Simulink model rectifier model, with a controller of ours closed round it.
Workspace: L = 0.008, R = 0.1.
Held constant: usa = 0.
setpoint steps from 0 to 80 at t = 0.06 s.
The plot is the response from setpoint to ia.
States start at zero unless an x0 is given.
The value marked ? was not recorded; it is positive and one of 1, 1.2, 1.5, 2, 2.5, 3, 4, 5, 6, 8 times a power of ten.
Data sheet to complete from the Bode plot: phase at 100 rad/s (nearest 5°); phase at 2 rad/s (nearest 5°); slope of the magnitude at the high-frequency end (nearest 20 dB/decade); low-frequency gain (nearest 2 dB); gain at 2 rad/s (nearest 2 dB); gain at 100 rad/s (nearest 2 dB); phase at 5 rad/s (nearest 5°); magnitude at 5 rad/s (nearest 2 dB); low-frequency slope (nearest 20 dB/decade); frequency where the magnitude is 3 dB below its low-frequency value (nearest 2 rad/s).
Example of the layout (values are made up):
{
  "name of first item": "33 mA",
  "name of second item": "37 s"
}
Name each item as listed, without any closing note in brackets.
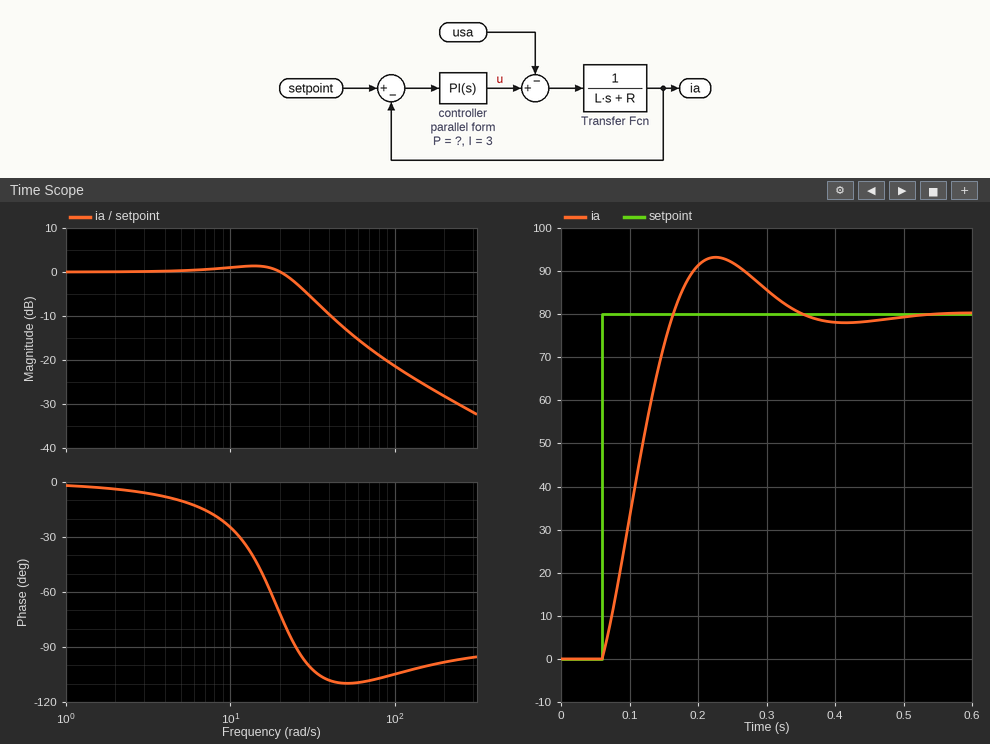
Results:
{
  "phase at 100 rad/s": "-105°",
  "phase at 2 rad/s": "-5°",
  "slope of the magnitude at the high-frequency end": "-20 dB/decade",
  "low-frequency gain": "0 dB",
  "gain at 2 rad/s": "0 dB",
  "gain at 100 rad/s": "-22 dB",
  "phase at 5 rad/s": "-10°",
  "magnitude at 5 rad/s": "0 dB",
  "low-frequency slope": "0 dB/decade",
  "frequency where the magnitude is 3 dB below its low-frequency value": "26 rad/s"
}
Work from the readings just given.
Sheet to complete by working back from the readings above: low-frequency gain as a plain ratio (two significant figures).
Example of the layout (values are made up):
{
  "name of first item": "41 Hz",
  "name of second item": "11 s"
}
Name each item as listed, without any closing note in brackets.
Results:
{
  "low-frequency gain as a plain ratio": "1.0"
}
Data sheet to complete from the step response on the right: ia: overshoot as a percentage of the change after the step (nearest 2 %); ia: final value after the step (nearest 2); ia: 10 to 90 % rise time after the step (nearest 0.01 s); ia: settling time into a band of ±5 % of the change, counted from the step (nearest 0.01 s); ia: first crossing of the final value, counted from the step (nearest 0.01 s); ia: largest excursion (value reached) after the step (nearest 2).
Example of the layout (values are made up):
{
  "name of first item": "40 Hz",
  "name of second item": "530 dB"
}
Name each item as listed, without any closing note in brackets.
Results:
{
  "ia: overshoot as a percentage of the change after the step": "16 %",
  "ia: final value after the step": "80",
  "ia: 10 to 90 % rise time after the step": "0.08 s",
  "ia: settling time into a band of ±5 % of the change, counted from the step": "0.25 s",
  "ia: first crossing of the final value, counted from the step": "0.10 s",
  "ia: largest excursion (value reached) after the step": "94"
}
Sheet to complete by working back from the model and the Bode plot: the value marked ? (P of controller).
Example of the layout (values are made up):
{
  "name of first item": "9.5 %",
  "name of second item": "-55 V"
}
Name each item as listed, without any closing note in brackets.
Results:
{
  "the value marked ?": "0.06"
}
